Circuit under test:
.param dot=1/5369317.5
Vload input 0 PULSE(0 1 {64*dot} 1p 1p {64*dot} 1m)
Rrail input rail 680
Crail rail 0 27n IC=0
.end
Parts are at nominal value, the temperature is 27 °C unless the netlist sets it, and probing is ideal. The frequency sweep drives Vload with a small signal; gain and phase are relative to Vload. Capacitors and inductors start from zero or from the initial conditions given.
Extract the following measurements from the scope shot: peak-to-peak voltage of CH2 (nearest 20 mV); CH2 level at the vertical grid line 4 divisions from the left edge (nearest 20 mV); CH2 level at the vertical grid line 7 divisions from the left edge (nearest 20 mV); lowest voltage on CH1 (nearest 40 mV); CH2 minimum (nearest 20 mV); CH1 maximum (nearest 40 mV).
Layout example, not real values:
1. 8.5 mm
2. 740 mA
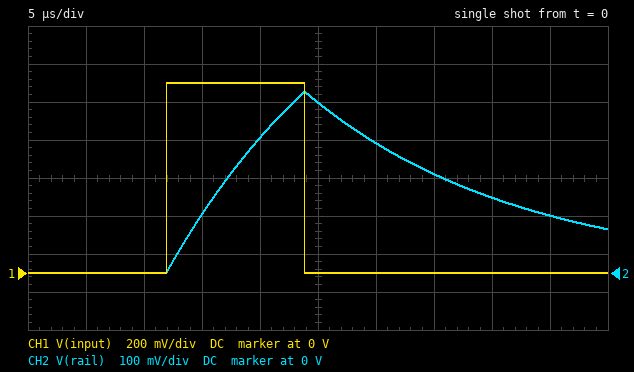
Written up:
1. 480 mV
2. 360 mV
3. 260 mV
4. 0 V
5. 0 V
6. 1.00 V
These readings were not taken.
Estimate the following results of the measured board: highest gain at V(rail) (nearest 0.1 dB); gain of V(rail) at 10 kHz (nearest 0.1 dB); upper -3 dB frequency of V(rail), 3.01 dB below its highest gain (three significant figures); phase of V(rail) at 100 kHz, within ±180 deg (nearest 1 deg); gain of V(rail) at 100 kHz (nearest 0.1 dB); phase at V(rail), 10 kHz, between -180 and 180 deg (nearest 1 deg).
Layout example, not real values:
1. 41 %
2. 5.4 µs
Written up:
1. 0 dB
2. -3.7 dB
3. 8.67 kHz
4. -85 deg
5. -21.3 dB
6. -49 deg
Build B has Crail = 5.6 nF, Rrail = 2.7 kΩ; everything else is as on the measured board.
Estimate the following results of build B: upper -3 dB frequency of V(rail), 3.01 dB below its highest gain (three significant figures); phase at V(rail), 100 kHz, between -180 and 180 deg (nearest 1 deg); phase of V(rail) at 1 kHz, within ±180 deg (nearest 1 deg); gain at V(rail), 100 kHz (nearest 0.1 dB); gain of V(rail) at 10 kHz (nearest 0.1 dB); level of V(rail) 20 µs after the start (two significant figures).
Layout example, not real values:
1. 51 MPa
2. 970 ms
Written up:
1. 10.5 kHz
2. -84 deg
3. -5 deg
4. -19.6 dB
5. -2.8 dB
6. 410 mV
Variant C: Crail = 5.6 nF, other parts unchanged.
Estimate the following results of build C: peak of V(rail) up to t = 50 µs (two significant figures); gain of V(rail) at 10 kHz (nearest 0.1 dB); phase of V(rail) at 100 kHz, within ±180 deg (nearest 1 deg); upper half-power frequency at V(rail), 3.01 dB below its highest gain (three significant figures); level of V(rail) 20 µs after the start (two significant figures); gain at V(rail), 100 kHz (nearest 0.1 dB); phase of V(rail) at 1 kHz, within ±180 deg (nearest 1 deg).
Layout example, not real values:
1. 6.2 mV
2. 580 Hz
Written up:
1. 960 mV
2. -0.2 dB
3. -67 deg
4. 41.8 kHz
5. 880 mV
6. -8.3 dB
7. -1 deg
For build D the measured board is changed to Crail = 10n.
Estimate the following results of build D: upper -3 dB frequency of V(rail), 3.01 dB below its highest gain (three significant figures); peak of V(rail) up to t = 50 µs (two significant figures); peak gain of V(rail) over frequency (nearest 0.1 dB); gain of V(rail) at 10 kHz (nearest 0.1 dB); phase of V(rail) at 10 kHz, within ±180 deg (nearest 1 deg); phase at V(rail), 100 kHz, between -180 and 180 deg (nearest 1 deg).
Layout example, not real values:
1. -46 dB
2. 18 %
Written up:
1. 23.4 kHz
2. 830 mV
3. 0 dB
4. -0.7 dB
5. -23 deg
6. -77 deg
